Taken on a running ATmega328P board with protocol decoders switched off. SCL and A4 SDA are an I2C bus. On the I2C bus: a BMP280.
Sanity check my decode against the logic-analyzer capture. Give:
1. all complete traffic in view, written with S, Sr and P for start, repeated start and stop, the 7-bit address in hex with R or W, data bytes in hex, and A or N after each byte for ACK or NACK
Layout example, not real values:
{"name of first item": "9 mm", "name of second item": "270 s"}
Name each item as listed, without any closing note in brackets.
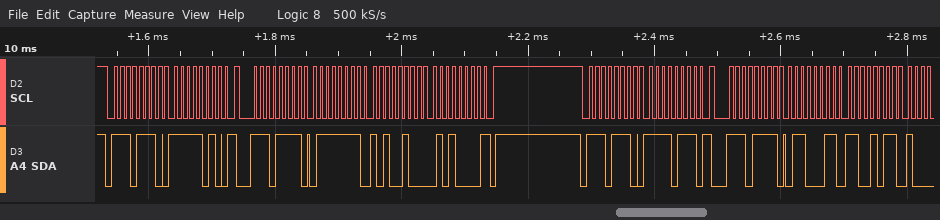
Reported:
{"all complete traffic in view, written with S, Sr and P for start, repeated start and stop, the 7-bit address in hex with R or W, data bytes in hex, and A or N after each byte for ACK or NACK": "S 77W A FA A Sr 77R A 7F A A4 A 50 N P S 77W A F7 A Sr 77R A 63 A CB A"}
